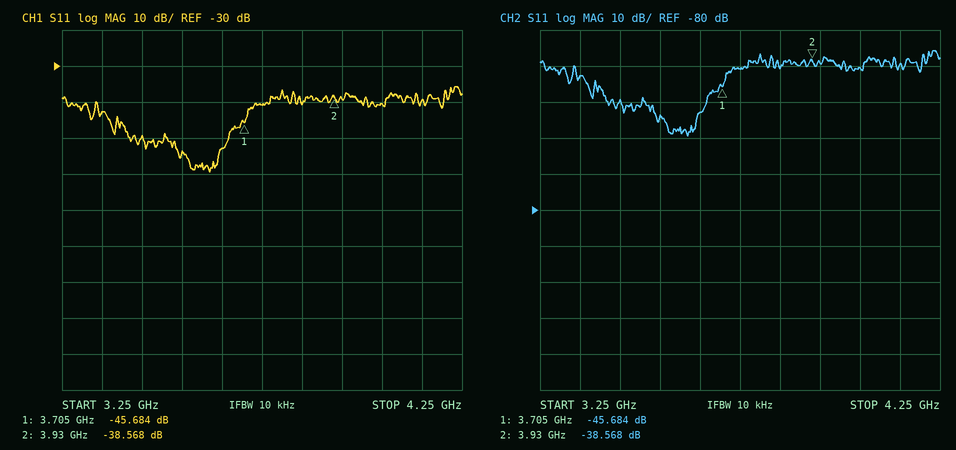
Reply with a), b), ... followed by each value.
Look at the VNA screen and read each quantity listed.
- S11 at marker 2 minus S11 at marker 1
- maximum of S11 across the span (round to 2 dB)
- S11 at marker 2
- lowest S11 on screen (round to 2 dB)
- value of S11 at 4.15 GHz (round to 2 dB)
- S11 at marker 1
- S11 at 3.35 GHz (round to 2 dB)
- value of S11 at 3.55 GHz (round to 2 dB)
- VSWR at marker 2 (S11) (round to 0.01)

a) 7.116 dB
b) -36 dB
c) -38.568 dB
d) -60 dB
e) -40 dB
f) -45.684 dB
g) -42 dB
h) -54 dB
i) 1.02
